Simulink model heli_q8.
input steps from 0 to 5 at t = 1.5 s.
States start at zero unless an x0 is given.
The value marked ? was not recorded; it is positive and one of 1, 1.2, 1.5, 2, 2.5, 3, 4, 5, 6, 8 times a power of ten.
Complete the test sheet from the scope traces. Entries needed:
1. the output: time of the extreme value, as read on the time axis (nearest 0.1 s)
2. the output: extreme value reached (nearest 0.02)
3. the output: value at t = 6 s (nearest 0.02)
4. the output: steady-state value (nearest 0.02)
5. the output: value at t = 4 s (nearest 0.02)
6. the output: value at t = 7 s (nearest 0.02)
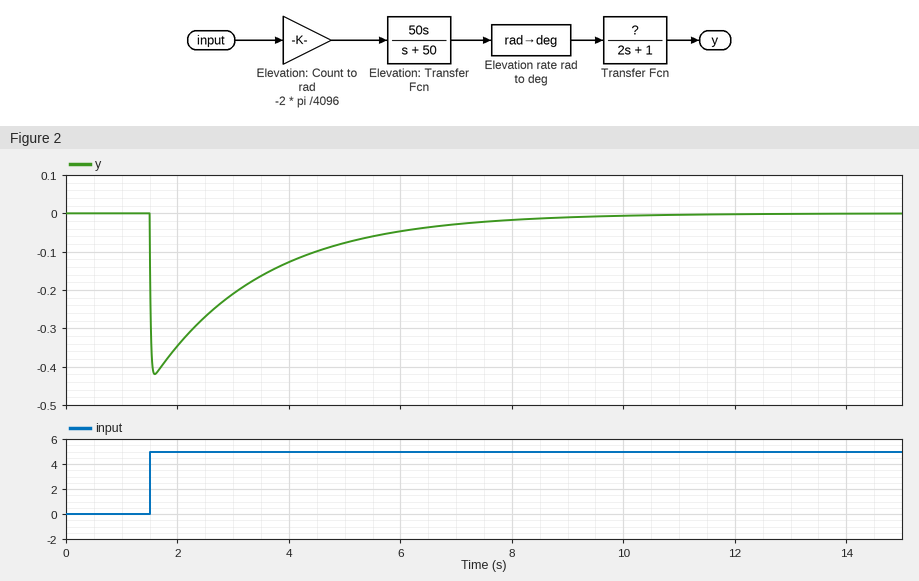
1.6 s
-0.42
-0.04
0.00
-0.12
-0.02
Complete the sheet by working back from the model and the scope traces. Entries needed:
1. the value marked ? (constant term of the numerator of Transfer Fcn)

2
